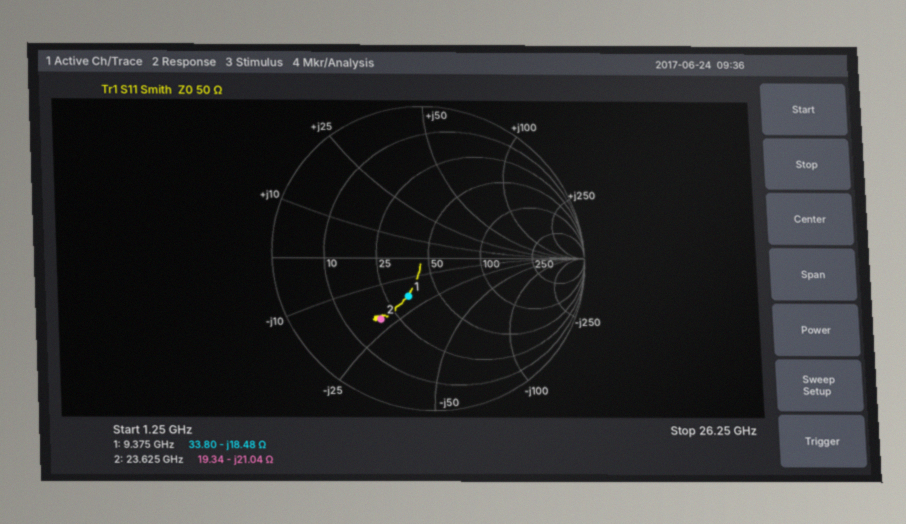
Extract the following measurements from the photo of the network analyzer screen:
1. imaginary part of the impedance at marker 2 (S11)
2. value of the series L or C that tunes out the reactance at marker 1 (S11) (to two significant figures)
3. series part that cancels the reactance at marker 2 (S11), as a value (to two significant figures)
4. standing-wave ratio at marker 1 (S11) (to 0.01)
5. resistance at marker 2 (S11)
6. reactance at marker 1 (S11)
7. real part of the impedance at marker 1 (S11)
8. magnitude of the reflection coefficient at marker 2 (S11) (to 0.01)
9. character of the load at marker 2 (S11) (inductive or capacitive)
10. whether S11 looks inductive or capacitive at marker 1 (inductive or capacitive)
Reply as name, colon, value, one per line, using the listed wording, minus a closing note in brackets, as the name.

imaginary part of the impedance at marker 2: -21.04 Ω
value of the series L or C that tunes out the reactance at marker 1 (S11): 310 pH
series part that cancels the reactance at marker 2 (S11), as a value: 140 pH
standing-wave ratio at marker 1 (S11): 1.80
resistance at marker 2: 19.34 Ω
reactance at marker 1: -18.48 Ω
real part of the impedance at marker 1: 33.80 Ω
magnitude of the reflection coefficient at marker 2 (S11): 0.51
character of the load at marker 2 (S11): capacitive
whether S11 looks inductive or capacitive at marker 1: capacitive
